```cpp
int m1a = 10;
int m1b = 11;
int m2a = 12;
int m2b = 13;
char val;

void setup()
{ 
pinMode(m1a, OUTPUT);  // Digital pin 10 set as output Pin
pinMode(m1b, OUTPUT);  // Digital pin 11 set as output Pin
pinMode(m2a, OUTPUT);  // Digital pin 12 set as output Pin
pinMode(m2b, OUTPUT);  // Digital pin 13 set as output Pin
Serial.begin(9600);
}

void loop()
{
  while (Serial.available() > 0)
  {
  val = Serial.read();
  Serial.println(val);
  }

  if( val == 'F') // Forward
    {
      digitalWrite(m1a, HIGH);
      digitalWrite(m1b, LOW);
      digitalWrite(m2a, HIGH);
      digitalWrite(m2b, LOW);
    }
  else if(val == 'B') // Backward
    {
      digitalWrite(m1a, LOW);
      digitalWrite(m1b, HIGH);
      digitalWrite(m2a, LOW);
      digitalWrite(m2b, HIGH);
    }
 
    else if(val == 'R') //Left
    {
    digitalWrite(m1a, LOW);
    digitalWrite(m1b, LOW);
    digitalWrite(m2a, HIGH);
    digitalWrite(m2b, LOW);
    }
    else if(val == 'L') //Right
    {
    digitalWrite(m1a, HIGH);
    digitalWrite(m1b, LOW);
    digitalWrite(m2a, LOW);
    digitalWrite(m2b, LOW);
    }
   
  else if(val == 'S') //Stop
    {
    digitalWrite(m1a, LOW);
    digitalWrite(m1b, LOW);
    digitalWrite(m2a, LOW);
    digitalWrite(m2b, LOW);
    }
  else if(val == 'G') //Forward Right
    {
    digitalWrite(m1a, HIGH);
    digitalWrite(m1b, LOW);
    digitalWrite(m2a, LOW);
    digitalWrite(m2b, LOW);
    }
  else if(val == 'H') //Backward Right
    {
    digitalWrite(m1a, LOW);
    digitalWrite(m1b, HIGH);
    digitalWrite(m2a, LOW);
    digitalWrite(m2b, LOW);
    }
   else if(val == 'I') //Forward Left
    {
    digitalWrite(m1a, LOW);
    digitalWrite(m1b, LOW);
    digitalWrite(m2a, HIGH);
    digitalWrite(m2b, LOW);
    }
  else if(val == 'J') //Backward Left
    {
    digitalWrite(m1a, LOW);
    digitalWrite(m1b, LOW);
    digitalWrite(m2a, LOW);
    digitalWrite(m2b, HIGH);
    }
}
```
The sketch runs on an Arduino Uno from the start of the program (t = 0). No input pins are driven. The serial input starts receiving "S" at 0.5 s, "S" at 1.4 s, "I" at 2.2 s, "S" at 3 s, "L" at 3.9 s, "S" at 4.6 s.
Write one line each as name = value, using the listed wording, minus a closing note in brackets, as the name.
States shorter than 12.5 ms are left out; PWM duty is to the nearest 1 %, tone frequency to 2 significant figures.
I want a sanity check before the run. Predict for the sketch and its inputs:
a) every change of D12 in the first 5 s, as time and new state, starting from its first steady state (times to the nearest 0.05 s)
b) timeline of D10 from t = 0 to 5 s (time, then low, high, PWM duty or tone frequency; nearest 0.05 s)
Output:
every change of D12 in the first 5 s, as time and new state, starting from its first steady state = 0 s low; 2.2 s high; 3 s low
timeline of D10 from t = 0 to 5 s = 0 s low; 3.9 s high; 4.6 s low
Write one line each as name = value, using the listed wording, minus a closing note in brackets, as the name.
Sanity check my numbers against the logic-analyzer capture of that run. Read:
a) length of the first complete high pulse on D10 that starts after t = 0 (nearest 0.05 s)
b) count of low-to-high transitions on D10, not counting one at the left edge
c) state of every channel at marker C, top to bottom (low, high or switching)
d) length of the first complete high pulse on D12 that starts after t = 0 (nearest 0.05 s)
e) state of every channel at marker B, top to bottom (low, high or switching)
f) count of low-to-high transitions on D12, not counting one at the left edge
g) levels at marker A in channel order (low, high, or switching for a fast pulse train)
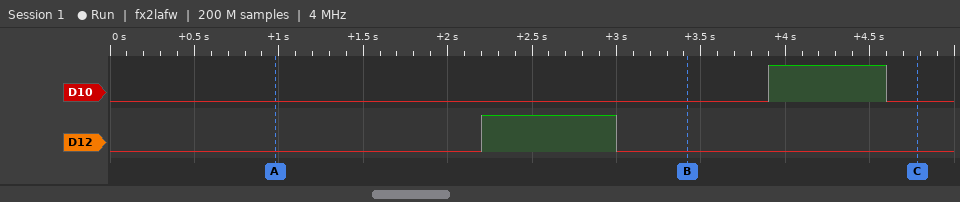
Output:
length of the first complete high pulse on D10 that starts after t = 0 = 0.70 s
count of low-to-high transitions on D10, not counting one at the left edge = 1
state of every channel at marker C, top to bottom = D10 low, D12 low
length of the first complete high pulse on D12 that starts after t = 0 = 0.80 s
state of every channel at marker B, top to bottom = D10 low, D12 low
count of low-to-high transitions on D12, not counting one at the left edge = 1
levels at marker A in channel order = D10 low, D12 low
